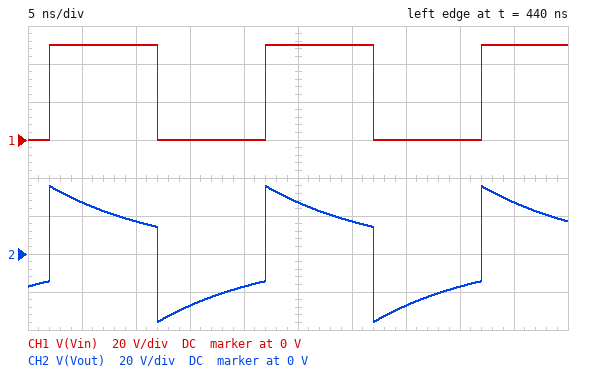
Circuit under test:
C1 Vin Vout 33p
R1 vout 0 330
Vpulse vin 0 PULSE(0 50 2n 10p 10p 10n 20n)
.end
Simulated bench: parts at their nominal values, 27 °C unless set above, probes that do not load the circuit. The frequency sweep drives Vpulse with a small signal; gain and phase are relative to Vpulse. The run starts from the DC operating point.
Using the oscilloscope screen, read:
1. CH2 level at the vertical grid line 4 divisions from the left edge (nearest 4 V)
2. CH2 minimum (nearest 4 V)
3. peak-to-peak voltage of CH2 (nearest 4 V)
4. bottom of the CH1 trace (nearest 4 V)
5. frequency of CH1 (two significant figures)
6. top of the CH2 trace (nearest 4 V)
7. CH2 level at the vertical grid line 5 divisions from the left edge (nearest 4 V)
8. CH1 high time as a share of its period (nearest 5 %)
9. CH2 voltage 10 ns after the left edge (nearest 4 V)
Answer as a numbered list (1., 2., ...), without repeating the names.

1. -16 V
2. -36 V
3. 72 V
4. 0 V
5. 50 MHz
6. 36 V
7. 28 V
8. 50 %
9. 16 V
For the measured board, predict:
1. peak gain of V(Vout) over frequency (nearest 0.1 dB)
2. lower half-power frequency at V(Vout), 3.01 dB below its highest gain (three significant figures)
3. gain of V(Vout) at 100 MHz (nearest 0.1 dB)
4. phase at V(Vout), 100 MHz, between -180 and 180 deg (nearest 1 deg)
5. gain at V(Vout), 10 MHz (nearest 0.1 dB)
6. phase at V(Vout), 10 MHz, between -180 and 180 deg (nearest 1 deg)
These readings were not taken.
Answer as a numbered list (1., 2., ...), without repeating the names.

1. 0 dB
2. 14.6 MHz
3. -0.1 dB
4. 8 deg
5. -5.0 dB
6. 56 deg
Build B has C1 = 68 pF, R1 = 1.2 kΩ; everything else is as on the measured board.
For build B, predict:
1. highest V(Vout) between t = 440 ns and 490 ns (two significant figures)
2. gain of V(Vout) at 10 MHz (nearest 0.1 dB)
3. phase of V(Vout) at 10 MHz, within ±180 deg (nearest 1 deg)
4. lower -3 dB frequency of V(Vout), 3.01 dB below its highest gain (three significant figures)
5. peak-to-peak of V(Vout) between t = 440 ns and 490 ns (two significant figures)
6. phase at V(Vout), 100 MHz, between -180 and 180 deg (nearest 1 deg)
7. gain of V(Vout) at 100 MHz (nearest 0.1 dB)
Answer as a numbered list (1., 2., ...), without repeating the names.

1. 27 V
2. -0.2 dB
3. 11 deg
4. 1.95 MHz
5. 53 V
6. 1 deg
7. 0 dB
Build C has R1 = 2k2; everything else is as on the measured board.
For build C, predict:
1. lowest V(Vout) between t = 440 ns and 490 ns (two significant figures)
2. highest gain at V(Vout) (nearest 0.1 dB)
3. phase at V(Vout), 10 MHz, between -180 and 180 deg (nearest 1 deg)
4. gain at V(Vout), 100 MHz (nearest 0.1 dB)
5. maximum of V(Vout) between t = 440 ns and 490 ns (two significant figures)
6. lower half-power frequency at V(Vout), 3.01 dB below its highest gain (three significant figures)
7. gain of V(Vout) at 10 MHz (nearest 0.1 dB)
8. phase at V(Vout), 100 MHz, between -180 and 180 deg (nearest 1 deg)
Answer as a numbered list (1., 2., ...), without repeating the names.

1. -27 V
2. 0 dB
3. 12 deg
4. 0 dB
5. 27 V
6. 2.19 MHz
7. -0.2 dB
8. 1 deg
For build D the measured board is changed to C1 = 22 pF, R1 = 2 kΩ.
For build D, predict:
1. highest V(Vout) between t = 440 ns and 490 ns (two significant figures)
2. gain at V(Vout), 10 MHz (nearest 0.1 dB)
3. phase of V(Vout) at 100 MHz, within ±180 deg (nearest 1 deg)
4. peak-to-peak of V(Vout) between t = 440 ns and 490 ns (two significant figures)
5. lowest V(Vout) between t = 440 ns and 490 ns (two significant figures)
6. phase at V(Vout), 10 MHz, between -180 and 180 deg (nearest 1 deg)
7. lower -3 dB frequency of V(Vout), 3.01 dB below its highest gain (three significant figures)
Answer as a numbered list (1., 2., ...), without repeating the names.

1. 28 V
2. -0.5 dB
3. 2 deg
4. 56 V
5. -28 V
6. 20 deg
7. 3.62 MHz
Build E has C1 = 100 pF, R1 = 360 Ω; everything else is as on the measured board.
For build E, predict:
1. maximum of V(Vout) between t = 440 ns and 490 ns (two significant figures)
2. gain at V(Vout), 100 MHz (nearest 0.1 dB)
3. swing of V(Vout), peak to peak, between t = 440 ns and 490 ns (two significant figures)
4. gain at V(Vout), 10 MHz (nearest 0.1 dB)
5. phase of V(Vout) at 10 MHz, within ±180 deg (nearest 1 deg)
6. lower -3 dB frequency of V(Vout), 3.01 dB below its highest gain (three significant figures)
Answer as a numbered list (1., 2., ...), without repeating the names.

1. 28 V
2. 0 dB
3. 57 V
4. -0.8 dB
5. 24 deg
6. 4.42 MHz
